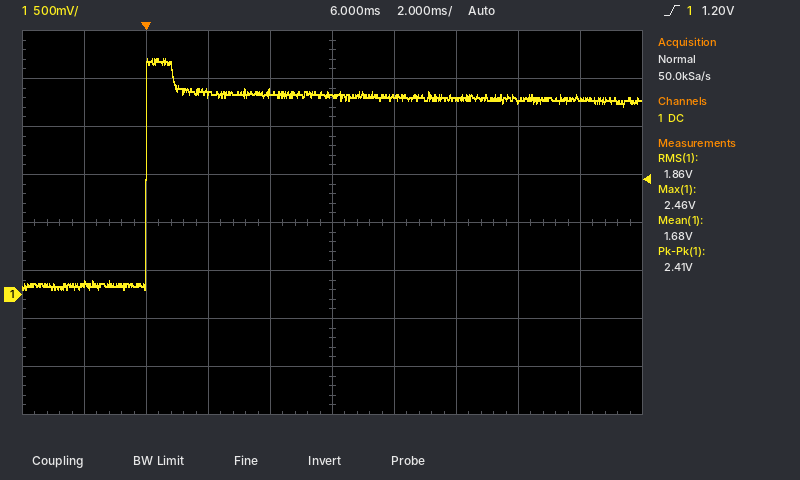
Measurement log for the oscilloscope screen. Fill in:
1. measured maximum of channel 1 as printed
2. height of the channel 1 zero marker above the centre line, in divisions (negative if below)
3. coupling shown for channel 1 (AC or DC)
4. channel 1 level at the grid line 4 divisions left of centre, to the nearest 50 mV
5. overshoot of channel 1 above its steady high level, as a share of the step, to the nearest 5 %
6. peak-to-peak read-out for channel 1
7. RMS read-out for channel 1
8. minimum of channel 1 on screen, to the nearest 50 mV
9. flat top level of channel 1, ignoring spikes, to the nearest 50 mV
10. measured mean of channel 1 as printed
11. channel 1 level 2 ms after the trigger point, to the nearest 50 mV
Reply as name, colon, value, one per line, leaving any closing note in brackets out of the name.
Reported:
measured maximum of channel 1 as printed: 2.46 V
height of the channel 1 zero marker above the centre line, in divisions: -1.5 div
coupling shown for channel 1: DC
channel 1 level at the grid line 4 divisions left of centre, to the nearest 50 mV: 100 mV
overshoot of channel 1 above its steady high level, as a share of the step, to the nearest 5 %: 20 %
peak-to-peak read-out for channel 1: 2.41 V
RMS read-out for channel 1: 1.86 V
minimum of channel 1 on screen, to the nearest 50 mV: 50 mV
flat top level of channel 1, ignoring spikes, to the nearest 50 mV: 2.05 V
measured mean of channel 1 as printed: 1.68 V
channel 1 level 2 ms after the trigger point, to the nearest 50 mV: 2.10 V
